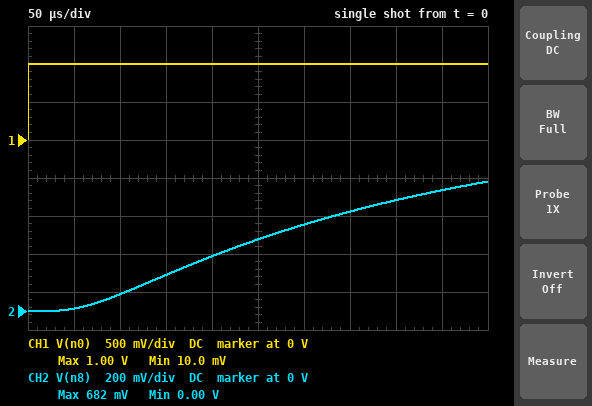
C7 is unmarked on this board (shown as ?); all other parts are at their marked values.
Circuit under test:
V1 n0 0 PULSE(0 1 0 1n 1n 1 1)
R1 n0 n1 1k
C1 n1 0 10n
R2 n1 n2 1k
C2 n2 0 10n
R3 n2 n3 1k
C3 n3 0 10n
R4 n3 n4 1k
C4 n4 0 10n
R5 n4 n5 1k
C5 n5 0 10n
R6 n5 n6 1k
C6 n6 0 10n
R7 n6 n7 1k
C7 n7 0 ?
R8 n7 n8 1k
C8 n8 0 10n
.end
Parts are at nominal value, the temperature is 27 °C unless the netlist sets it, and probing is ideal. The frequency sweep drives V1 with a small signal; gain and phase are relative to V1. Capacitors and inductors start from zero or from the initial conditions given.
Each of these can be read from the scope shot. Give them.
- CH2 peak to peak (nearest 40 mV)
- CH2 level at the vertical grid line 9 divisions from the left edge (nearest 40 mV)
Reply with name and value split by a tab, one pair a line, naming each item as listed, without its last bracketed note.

CH2 peak to peak	680 mV
CH2 level at the vertical grid line 9 divisions from the left edge	640 mV
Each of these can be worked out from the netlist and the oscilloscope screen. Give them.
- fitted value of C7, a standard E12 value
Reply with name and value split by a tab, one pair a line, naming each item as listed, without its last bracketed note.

fitted value of C7, a standard E12 value	22 nF
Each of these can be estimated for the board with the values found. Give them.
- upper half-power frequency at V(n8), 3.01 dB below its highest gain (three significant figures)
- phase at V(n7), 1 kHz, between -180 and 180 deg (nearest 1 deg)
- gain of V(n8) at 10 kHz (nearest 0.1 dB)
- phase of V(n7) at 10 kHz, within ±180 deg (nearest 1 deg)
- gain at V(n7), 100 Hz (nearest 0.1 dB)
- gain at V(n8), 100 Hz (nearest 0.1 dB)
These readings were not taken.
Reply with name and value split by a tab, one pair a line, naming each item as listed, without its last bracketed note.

upper half-power frequency at V(n8), 3.01 dB below its highest gain	423 Hz
phase at V(n7), 1 kHz, between -180 and 180 deg	-89 deg
gain of V(n8) at 10 kHz	-39.4 dB
phase of V(n7) at 10 kHz, within ±180 deg	122 deg
gain at V(n7), 100 Hz	-0.2 dB
gain at V(n8), 100 Hz	-0.2 dB
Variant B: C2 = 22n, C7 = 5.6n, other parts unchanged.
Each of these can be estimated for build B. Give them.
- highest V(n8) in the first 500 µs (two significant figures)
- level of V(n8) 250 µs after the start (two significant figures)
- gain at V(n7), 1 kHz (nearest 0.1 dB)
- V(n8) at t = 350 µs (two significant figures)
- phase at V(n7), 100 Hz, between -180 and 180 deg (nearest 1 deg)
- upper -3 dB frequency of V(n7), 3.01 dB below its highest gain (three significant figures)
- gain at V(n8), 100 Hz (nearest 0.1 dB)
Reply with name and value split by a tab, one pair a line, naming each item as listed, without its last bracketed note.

highest V(n8) in the first 500 µs	780 mV
level of V(n8) 250 µs after the start	460 mV
gain at V(n7), 1 kHz	-6.4 dB
V(n8) at t = 350 µs	620 mV
phase at V(n7), 100 Hz, between -180 and 180 deg	-12 deg
upper -3 dB frequency of V(n7), 3.01 dB below its highest gain	560 Hz
gain at V(n8), 100 Hz	-0.1 dB
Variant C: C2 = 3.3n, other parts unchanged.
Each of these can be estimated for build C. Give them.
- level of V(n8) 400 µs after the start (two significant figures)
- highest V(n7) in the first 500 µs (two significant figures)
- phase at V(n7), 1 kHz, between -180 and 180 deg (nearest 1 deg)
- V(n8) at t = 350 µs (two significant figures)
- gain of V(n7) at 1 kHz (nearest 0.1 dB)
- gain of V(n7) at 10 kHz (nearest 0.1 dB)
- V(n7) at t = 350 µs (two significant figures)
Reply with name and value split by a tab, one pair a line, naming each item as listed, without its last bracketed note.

level of V(n8) 400 µs after the start	600 mV
highest V(n7) in the first 500 µs	700 mV
phase at V(n7), 1 kHz, between -180 and 180 deg	-86 deg
V(n8) at t = 350 µs	540 mV
gain of V(n7) at 1 kHz	-8.2 dB
gain of V(n7) at 10 kHz	-36.3 dB
V(n7) at t = 350 µs	550 mV
